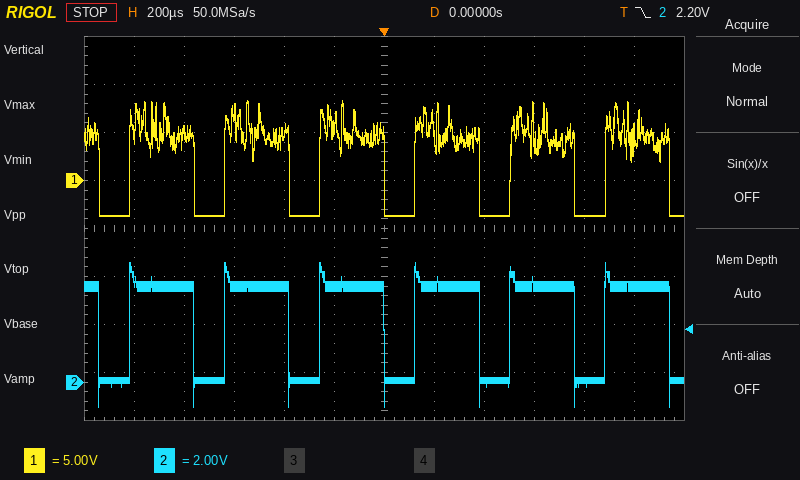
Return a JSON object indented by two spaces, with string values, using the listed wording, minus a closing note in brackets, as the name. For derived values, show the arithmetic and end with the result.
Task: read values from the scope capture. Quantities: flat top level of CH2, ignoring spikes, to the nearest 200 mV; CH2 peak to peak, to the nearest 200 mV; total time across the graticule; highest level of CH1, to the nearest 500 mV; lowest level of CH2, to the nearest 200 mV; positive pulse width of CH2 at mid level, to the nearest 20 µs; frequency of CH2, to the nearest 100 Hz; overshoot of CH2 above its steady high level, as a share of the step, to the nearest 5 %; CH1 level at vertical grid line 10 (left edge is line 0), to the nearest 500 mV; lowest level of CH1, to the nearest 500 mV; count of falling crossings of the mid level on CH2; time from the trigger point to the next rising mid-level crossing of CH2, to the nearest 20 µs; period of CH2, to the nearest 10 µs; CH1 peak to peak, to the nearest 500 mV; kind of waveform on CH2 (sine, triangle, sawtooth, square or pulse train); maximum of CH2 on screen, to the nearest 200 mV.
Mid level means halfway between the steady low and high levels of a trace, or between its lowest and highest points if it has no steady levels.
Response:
{
  "flat top level of CH2, ignoring spikes, to the nearest 200 mV": "4.0 V",
  "CH2 peak to peak, to the nearest 200 mV": "5.0 V − (-1.0 V) = 6.0 V",
  "total time across the graticule": "2.4 ms",
  "highest level of CH1, to the nearest 500 mV": "8.5 V",
  "lowest level of CH2, to the nearest 200 mV": "-1.0 V",
  "positive pulse width of CH2 at mid level, to the nearest 20 µs": "260 µs",
  "frequency of CH2, to the nearest 100 Hz": "1 / 380 µs ≈ 2.6 kHz",
  "overshoot of CH2 above its steady high level, as a share of the step, to the nearest 5 %": "25 %",
  "CH1 level at vertical grid line 10 (left edge is line 0), to the nearest 500 mV": "-3.5 V",
  "lowest level of CH1, to the nearest 500 mV": "-3.5 V",
  "count of falling crossings of the mid level on CH2": "7",
  "time from the trigger point to the next rising mid-level crossing of CH2, to the nearest 20 µs": "120 µs",
  "period of CH2, to the nearest 10 µs": "380 µs",
  "CH1 peak to peak, to the nearest 500 mV": "8.5 V − (-3.5 V) = 12.0 V",
  "kind of waveform on CH2": "pulse train",
  "maximum of CH2 on screen, to the nearest 200 mV": "5.0 V"
}
